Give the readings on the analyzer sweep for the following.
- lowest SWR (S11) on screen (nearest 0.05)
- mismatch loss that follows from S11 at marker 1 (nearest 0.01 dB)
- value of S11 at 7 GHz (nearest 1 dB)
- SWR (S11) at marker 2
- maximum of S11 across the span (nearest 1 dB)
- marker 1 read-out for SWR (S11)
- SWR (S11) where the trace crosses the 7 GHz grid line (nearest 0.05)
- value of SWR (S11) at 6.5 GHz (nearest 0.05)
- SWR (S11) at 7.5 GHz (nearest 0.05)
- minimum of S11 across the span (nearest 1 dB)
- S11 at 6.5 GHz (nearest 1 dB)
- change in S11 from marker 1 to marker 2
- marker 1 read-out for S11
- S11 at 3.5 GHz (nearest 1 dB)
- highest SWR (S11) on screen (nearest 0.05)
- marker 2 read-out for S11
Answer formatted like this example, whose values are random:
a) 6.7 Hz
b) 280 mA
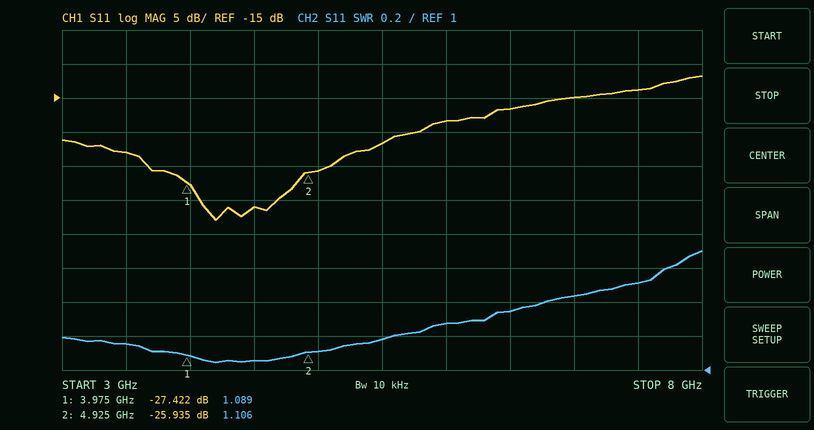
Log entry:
a) 1.05
b) 0.01 dB
c) -15 dB
d) 1.106
e) -12 dB
f) 1.089
g) 1.45
h) 1.35
i) 1.50
j) -33 dB
k) -17 dB
l) 1.487 dB
m) -27.422 dB
n) -23 dB
o) 1.70
p) -25.935 dB
